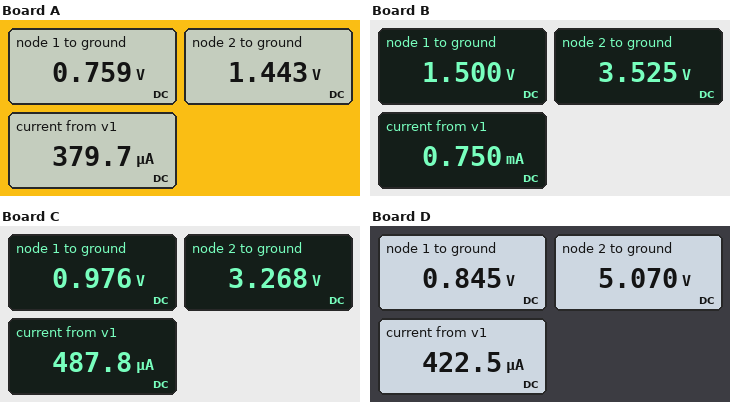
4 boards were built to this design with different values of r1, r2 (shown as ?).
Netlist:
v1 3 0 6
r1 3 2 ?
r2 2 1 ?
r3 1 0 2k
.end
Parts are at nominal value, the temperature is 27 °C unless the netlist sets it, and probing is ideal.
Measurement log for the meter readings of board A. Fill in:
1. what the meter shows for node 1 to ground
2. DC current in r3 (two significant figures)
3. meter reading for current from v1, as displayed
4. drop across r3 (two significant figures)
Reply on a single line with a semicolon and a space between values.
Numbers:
0.759 V; 380 µA; 379.7 µA; 760 mV
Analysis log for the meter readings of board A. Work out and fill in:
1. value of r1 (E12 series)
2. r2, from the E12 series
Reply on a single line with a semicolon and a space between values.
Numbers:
12 kΩ; 1.8 kΩ
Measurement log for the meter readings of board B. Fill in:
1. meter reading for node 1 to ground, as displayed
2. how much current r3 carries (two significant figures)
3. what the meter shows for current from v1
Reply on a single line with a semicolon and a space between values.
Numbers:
1.500 V; 750 µA; 0.750 mA
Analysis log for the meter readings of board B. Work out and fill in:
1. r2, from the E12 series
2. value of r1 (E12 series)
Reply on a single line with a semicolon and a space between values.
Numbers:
2.7 kΩ; 3.3 kΩ
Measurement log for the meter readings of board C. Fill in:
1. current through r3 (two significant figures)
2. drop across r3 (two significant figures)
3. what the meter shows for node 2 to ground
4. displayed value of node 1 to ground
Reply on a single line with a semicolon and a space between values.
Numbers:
490 µA; 980 mV; 3.268 V; 0.976 V
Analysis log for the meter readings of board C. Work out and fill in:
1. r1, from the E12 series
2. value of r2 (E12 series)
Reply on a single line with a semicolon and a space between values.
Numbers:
5.6 kΩ; 4.7 kΩ
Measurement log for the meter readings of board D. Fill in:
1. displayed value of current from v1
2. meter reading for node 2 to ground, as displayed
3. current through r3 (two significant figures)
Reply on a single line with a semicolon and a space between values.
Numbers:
422.5 µA; 5.070 V; 420 µA
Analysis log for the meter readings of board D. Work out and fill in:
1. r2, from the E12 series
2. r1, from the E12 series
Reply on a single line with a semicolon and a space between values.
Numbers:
10 kΩ; 2.2 kΩ
